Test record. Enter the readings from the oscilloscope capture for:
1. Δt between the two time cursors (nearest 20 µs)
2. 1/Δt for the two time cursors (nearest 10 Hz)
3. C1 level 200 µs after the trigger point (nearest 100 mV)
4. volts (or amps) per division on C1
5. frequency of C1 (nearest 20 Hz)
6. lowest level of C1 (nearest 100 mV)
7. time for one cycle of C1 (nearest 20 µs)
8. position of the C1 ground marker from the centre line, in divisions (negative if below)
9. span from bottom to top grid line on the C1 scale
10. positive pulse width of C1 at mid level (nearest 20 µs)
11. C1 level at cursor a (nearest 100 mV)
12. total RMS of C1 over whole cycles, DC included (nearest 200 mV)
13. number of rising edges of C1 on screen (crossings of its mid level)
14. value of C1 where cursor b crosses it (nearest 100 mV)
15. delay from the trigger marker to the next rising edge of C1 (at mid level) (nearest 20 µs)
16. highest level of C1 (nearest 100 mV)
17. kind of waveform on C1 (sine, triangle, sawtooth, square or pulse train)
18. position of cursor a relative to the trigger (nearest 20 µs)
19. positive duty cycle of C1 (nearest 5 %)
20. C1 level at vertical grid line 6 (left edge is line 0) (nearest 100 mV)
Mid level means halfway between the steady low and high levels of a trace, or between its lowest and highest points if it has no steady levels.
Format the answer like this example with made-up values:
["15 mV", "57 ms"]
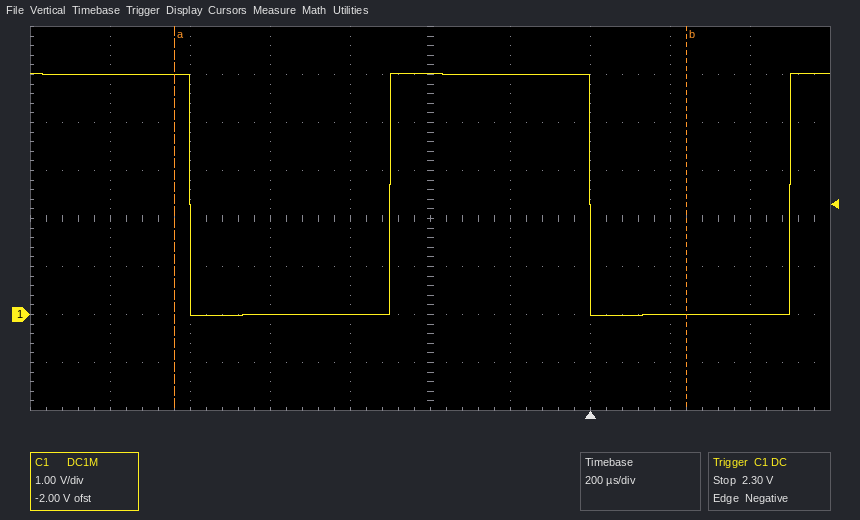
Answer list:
["1.28 ms", "780 Hz", "0.0 V", "1 V", "1.00 kHz", "0.0 V", "1.00 ms", "-2.0 div", "8 V", "500 µs", "5.0 V", "3.6 V", "2", "0.0 V", "500 µs", "5.0 V", "square", "-1.04 ms", "50 %", "5.0 V"]
